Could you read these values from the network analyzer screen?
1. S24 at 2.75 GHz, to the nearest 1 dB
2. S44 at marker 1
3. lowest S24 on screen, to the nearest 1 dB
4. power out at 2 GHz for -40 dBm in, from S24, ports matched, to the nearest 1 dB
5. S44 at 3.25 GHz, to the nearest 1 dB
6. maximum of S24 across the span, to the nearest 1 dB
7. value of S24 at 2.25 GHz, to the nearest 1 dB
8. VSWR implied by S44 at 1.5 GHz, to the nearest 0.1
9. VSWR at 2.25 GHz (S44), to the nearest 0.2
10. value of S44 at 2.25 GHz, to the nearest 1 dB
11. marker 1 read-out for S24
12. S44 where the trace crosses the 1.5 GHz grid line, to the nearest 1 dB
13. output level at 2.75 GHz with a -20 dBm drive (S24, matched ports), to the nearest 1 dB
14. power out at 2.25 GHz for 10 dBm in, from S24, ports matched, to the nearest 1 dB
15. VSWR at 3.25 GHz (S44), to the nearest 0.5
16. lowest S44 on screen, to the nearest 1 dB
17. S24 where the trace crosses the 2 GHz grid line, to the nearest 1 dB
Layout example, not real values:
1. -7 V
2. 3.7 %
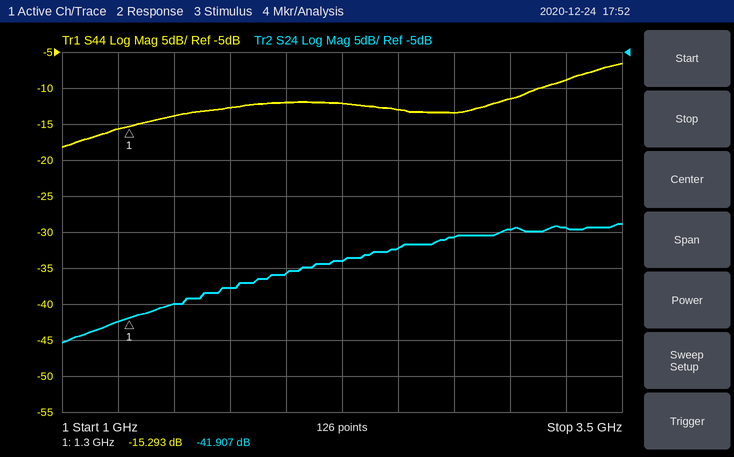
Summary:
1. -31 dB
2. -15.293 dB
3. -45 dB
4. -76 dBm
5. -9 dB
6. -29 dB
7. -34 dB
8. 1.5
9. 1.6
10. -12 dB
11. -41.907 dB
12. -14 dB
13. -51 dBm
14. -24 dBm
15. 2.0
16. -18 dB
17. -36 dB
